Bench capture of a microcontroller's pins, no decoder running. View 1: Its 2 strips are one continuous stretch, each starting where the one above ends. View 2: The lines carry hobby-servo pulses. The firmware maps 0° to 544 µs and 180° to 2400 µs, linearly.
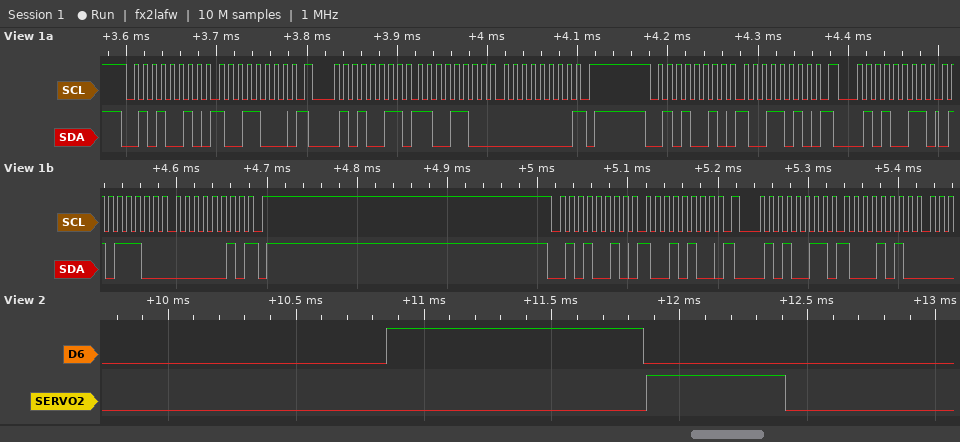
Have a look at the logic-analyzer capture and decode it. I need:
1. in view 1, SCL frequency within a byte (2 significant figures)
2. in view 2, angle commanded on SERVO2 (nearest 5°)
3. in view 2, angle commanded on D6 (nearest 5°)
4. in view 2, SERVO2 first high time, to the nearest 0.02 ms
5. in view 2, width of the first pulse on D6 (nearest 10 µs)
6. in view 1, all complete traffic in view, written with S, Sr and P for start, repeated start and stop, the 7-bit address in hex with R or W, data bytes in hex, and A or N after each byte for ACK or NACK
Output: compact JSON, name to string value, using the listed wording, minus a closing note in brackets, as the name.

{"in view 1, SCL frequency within a byte": "100 kHz", "in view 2, angle commanded on SERVO2": "0°", "in view 2, angle commanded on D6": "45°", "in view 2, SERVO2 first high time, to the nearest 0.02 ms": "0.54 ms", "in view 2, width of the first pulse on D6": "1010 µs", "in view 1, all complete traffic in view, written with S, Sr and P for start, repeated start and stop, the 7-bit address in hex with R or W, data bytes in hex, and A or N after each byte for ACK or NACK": "S 29W A 98 A Sr 29R A CC A 00 N P S 29W A 9A A Sr 29R A 5C A 02 N P S 29W A 94 A Sr 29R A 8A A"}
